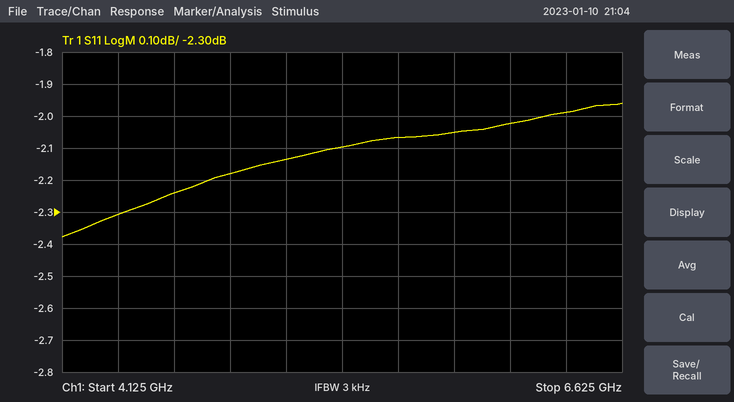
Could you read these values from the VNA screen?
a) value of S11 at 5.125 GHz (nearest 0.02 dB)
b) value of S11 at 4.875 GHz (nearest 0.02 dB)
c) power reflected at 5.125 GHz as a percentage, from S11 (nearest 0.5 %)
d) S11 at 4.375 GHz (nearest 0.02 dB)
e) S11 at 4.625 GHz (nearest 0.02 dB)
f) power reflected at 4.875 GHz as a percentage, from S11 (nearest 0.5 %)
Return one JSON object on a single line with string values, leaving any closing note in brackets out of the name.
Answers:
{"value of S11 at 5.125 GHz": "-2.14 dB", "value of S11 at 4.875 GHz": "-2.18 dB", "power reflected at 5.125 GHz as a percentage, from S11": "61.0 %", "S11 at 4.375 GHz": "-2.30 dB", "S11 at 4.625 GHz": "-2.24 dB", "power reflected at 4.875 GHz as a percentage, from S11": "60.5 %"}
